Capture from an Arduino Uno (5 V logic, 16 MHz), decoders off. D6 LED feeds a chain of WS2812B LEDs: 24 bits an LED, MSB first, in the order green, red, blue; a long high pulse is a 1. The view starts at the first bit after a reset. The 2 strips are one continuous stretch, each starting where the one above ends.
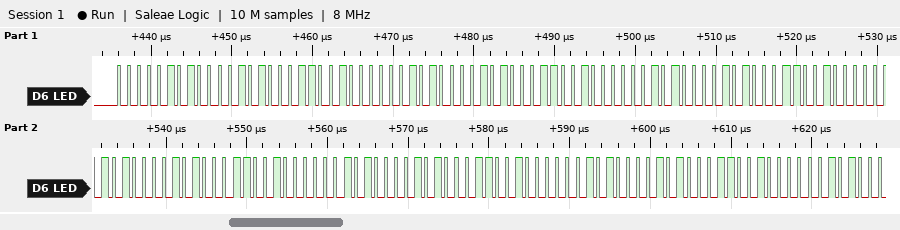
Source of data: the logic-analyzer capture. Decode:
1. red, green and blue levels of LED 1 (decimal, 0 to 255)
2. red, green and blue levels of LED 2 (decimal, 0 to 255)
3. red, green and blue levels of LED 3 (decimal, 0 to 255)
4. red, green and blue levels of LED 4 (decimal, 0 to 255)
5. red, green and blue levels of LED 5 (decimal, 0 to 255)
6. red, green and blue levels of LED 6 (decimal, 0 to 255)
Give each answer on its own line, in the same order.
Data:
10, 5, 50
10, 5, 50
10, 5, 50
10, 5, 50
10, 5, 50
10, 5, 50
